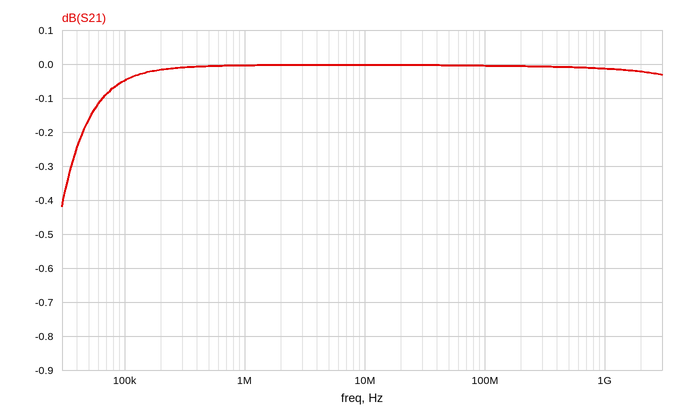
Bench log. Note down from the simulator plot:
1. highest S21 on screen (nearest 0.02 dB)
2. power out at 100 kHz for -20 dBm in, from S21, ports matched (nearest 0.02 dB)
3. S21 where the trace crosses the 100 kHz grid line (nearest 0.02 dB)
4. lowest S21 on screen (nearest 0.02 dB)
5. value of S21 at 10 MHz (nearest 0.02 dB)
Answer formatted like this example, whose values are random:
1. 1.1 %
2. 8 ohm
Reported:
1. 0.00 dB
2. -20.04 dBm
3. -0.04 dB
4. -0.42 dB
5. 0.00 dB
